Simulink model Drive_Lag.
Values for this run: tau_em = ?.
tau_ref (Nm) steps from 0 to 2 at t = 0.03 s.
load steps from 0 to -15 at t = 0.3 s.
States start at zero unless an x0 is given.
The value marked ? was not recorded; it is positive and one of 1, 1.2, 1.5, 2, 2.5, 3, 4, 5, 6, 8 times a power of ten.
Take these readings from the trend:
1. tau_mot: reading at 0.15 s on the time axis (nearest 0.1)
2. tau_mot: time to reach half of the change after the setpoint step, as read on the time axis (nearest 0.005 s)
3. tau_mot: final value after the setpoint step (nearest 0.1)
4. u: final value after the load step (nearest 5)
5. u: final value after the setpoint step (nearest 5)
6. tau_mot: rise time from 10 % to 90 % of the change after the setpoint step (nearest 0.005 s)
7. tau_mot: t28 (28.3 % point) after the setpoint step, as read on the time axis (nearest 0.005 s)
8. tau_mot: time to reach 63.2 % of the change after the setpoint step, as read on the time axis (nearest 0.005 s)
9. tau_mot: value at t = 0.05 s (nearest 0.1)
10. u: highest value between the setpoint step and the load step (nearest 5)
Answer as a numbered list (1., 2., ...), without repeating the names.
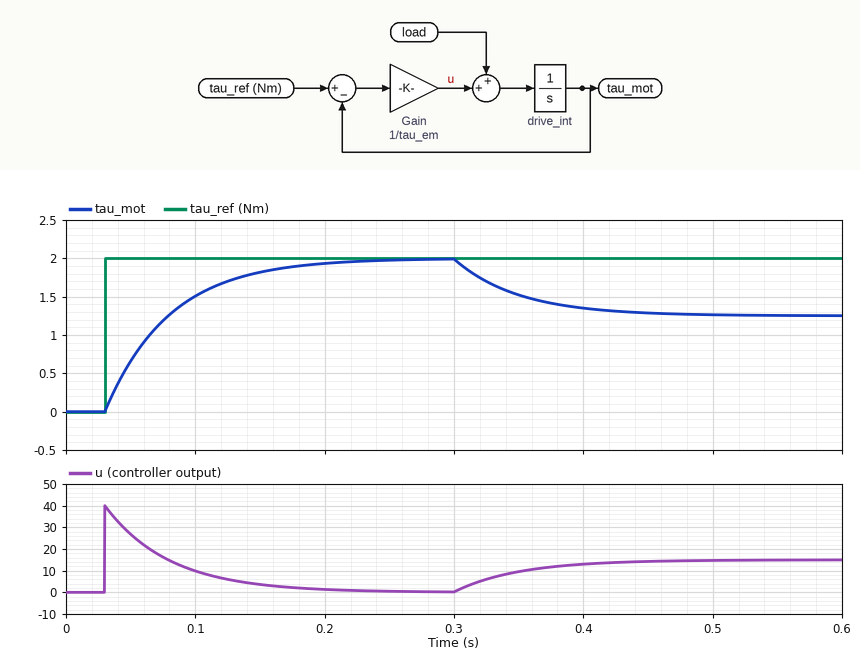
1. 1.8
2. 0.065 s
3. 2.0
4. 15
5. 0
6. 0.110 s
7. 0.045 s
8. 0.080 s
9. 0.7
10. 40
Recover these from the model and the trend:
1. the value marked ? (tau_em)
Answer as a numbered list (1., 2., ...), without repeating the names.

1. 0.05
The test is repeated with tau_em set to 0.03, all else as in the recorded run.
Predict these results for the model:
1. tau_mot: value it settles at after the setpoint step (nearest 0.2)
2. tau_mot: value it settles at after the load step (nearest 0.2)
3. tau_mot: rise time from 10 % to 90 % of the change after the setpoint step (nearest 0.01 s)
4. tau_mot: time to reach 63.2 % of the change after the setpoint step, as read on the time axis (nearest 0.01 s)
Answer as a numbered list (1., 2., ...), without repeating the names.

1. 2.0
2. 1.6
3. 0.07 s
4. 0.06 s
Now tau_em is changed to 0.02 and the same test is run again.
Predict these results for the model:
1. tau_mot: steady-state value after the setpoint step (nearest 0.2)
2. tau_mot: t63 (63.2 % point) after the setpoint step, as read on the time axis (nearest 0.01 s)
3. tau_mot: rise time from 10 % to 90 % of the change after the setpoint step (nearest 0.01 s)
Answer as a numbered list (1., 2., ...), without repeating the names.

1. 2.0
2. 0.05 s
3. 0.04 s
